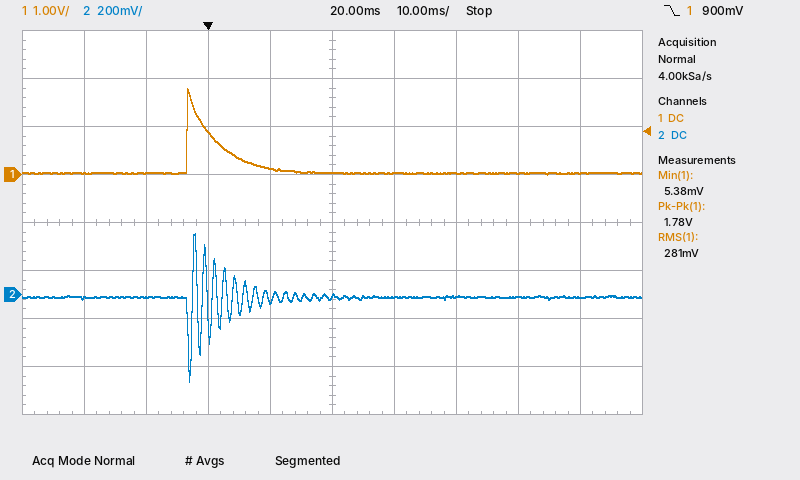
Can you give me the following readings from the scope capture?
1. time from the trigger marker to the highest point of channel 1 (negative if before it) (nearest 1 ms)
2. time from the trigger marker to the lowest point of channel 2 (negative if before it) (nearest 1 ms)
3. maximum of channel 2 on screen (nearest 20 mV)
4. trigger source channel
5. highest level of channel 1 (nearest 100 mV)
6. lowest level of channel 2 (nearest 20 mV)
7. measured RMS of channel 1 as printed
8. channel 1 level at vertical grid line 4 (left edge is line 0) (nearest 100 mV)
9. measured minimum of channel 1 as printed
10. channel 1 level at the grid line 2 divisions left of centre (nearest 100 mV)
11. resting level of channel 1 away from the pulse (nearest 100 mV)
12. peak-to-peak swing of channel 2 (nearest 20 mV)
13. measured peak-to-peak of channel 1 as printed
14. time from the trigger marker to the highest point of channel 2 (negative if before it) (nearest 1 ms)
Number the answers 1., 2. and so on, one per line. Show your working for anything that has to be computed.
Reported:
1. -3 ms
2. -3 ms
3. 260 mV
4. channel 1
5. 1.8 V
6. -360 mV
7. 281 mV
8. 100 mV
9. 5.38 mV
10. 900 mV
11. 0.0 V
12. 260 mV − (-360 mV) = 620 mV
13. 1.78 V
14. -2 ms
